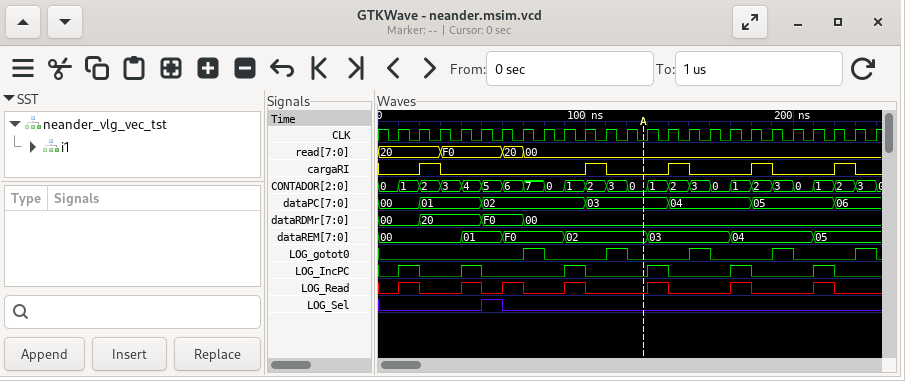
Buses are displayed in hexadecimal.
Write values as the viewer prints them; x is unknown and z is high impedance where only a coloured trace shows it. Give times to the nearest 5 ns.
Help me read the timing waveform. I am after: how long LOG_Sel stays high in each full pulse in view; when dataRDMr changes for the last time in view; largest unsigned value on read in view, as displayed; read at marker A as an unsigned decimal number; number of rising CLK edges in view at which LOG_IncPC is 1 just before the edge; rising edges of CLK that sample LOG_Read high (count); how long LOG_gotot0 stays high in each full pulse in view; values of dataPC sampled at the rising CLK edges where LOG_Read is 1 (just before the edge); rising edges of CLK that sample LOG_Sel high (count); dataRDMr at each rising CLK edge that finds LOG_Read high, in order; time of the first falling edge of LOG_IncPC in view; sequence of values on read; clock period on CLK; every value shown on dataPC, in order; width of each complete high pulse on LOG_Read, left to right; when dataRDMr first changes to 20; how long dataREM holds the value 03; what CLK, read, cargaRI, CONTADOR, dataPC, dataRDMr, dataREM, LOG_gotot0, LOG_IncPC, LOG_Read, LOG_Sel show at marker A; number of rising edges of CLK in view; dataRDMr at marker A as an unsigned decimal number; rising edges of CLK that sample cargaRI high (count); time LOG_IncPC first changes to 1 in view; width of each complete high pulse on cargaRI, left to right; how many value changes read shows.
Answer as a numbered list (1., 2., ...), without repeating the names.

1. 10 ns
2. 70 ns
3. F0
4. 0
5. 6
6. 7
7. 10 ns, 10 ns, 10 ns, 10 ns, 10 ns
8. 00, 01, 02, 02, 03, 04, 05
9. 1
10. 00, 20, F0, 00, 00, 00, 00
11. 20 ns
12. 20, F0, 20, 00
13. 10 ns
14. 00, 01, 02, 03, 04, 05, 06
15. 10 ns, 10 ns, 10 ns, 10 ns, 10 ns, 10 ns, 10 ns
16. 20 ns
17. 40 ns
18. CLK=0, read=00, cargaRI=0, CONTADOR=0, dataPC=03, dataRDMr=00, dataREM=02, LOG_gotot0=0, LOG_IncPC=0, LOG_Read=0, LOG_Sel=0
19. 24
20. 0
21. 5
22. 10 ns
23. 10 ns, 10 ns, 10 ns, 10 ns, 10 ns
24. 3
